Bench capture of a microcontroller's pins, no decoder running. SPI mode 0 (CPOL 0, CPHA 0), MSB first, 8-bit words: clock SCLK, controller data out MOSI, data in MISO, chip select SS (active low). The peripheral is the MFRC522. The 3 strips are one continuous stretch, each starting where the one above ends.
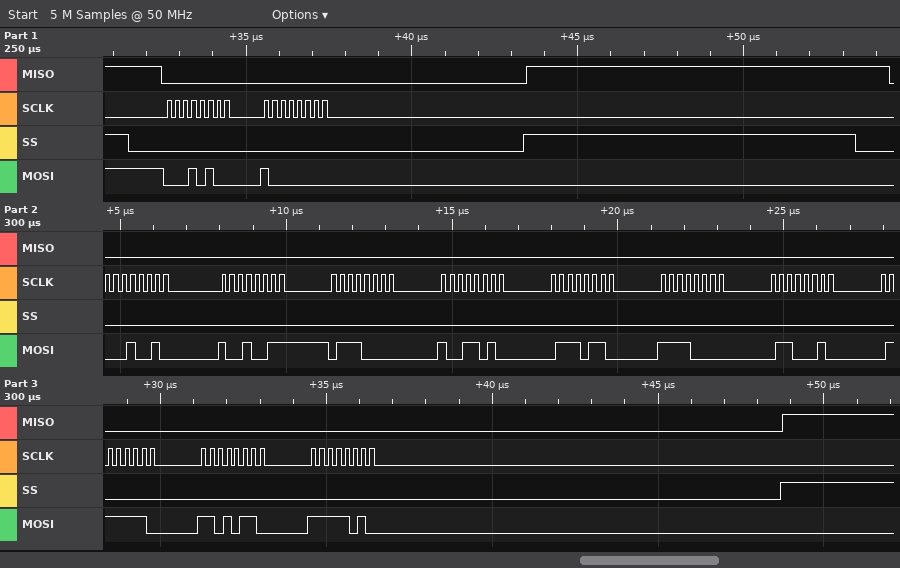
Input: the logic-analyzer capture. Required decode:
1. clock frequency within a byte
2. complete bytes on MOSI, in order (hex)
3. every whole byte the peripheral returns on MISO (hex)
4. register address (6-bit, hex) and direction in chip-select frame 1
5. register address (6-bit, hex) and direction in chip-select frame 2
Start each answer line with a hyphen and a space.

- 4 MHz
- 14 80 12 93 70 9A 76 F0 62 7E D6 FA
- 00 00 00 00 00 00 00 00 00 00 00 00
- 0x0A write
- 0x09 write
